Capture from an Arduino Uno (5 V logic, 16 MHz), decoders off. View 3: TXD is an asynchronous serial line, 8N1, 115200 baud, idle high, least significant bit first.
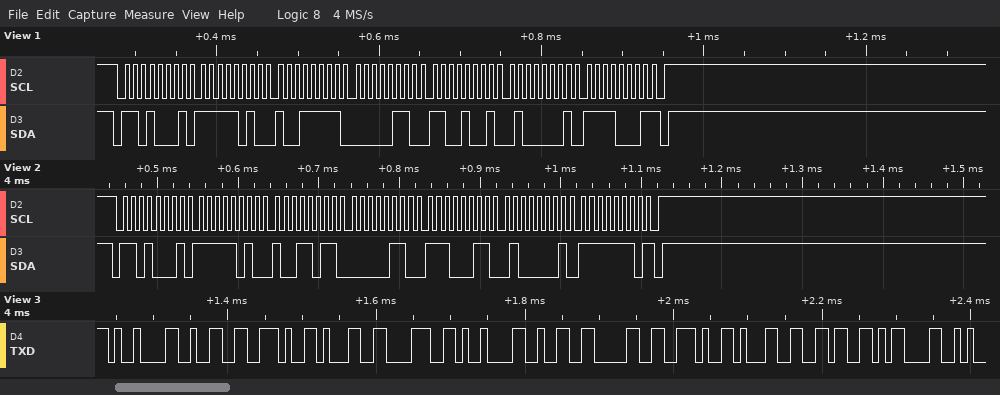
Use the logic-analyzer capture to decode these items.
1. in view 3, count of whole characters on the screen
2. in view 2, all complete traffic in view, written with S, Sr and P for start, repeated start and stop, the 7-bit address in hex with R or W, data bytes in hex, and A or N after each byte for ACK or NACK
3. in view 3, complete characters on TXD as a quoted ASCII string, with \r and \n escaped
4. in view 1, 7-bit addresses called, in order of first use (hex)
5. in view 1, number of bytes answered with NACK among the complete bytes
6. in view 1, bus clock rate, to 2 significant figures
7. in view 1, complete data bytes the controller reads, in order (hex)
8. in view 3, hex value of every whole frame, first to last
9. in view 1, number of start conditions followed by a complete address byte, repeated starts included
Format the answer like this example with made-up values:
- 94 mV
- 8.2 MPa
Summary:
- 12
- S 68R A FA A 9B A 06 A E3 A 41 A FE N P
- "\t2.18\t20.16\r"
- 0x68
- 1
- 100 kHz
- FA 9F 06 C9 41 F1
- 0x09 0x32 0x2E 0x31 0x38 0x09 0x32 0x30 0x2E 0x31 0x36 0x0D
- 1
